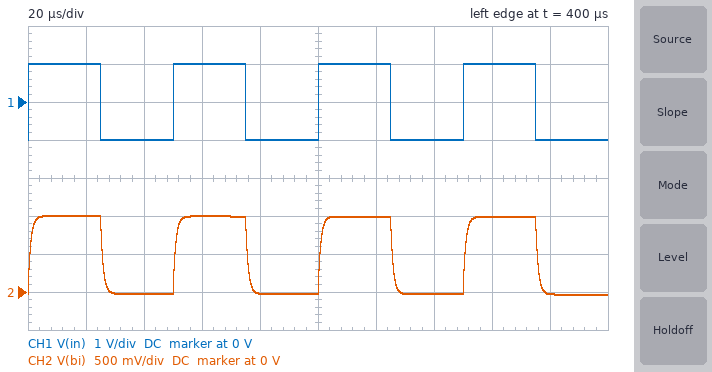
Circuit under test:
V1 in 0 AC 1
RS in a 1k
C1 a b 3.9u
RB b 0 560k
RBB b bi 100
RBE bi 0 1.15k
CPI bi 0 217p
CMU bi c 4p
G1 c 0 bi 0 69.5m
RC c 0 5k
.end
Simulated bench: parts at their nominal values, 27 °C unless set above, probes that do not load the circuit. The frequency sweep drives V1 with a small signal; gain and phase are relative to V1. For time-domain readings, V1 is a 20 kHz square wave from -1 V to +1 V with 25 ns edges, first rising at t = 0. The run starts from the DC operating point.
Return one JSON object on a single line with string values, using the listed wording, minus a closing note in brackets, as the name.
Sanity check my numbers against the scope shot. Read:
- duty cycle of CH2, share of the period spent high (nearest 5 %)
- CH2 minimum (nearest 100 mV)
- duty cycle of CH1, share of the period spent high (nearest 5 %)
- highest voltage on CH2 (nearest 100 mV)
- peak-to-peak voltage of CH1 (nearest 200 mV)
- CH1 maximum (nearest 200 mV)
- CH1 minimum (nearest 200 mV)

{"duty cycle of CH2, share of the period spent high": "50 %", "CH2 minimum": "0 V", "duty cycle of CH1, share of the period spent high": "50 %", "highest voltage on CH2": "1.0 V", "peak-to-peak voltage of CH1": "2.0 V", "CH1 maximum": "1.0 V", "CH1 minimum": "-1.0 V"}
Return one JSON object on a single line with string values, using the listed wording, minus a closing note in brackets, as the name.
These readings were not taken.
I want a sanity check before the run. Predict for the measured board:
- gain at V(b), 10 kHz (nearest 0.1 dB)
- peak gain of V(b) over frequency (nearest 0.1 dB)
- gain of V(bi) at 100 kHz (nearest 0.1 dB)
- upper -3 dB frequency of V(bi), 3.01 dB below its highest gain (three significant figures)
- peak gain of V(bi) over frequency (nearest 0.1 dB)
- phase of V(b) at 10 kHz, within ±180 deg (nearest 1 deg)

{"gain at V(b), 10 kHz": "-5.1 dB", "peak gain of V(b) over frequency": "-5.1 dB", "gain of V(bi) at 100 kHz": "-7.1 dB", "upper -3 dB frequency of V(bi), 3.01 dB below its highest gain": "173 kHz", "peak gain of V(bi) over frequency": "-5.8 dB", "phase of V(b) at 10 kHz, within ±180 deg": "-3 deg"}
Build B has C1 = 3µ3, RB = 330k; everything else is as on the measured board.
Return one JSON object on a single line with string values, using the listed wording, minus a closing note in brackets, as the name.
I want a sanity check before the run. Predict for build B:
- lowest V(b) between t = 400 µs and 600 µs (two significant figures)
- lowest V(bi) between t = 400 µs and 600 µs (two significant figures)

{"lowest V(b) between t = 400 µs and 600 µs": "-43 mV", "lowest V(bi) between t = 400 µs and 600 µs": "-40 mV"}
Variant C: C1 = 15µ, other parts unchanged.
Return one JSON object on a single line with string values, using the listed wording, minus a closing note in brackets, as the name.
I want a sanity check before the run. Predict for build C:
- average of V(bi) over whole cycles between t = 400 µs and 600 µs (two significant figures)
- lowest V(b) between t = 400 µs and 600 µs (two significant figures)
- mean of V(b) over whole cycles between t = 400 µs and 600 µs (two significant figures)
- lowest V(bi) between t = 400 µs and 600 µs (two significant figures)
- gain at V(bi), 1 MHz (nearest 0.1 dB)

{"average of V(bi) over whole cycles between t = 400 µs and 600 µs": "500 mV", "lowest V(b) between t = 400 µs and 600 µs": "-9.8 mV", "mean of V(b) over whole cycles between t = 400 µs and 600 µs": "550 mV", "lowest V(bi) between t = 400 µs and 600 µs": "-9.0 mV", "gain at V(bi), 1 MHz": "-21.2 dB"}
